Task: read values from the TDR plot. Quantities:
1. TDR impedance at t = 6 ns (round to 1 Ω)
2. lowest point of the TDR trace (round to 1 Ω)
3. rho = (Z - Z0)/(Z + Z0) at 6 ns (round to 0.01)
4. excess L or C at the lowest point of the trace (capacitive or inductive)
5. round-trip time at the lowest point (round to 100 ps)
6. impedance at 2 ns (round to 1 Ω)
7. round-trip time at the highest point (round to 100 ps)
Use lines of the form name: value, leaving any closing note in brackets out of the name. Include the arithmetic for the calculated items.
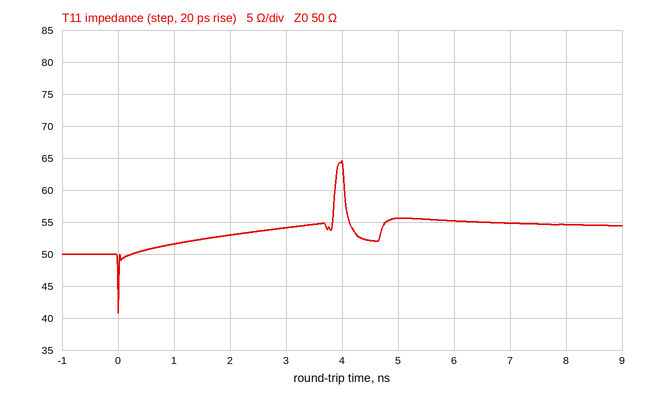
TDR impedance at t = 6 ns: 55 Ω
lowest point of the TDR trace: 41 Ω
rho = (Z - Z0)/(Z + Z0) at 6 ns: (55 − 50)/(55 + 50) ≈ +0.05
excess L or C at the lowest point of the trace: capacitive
round-trip time at the lowest point: 0.0 ns
impedance at 2 ns: 53 Ω
round-trip time at the highest point: 4.0 ns
